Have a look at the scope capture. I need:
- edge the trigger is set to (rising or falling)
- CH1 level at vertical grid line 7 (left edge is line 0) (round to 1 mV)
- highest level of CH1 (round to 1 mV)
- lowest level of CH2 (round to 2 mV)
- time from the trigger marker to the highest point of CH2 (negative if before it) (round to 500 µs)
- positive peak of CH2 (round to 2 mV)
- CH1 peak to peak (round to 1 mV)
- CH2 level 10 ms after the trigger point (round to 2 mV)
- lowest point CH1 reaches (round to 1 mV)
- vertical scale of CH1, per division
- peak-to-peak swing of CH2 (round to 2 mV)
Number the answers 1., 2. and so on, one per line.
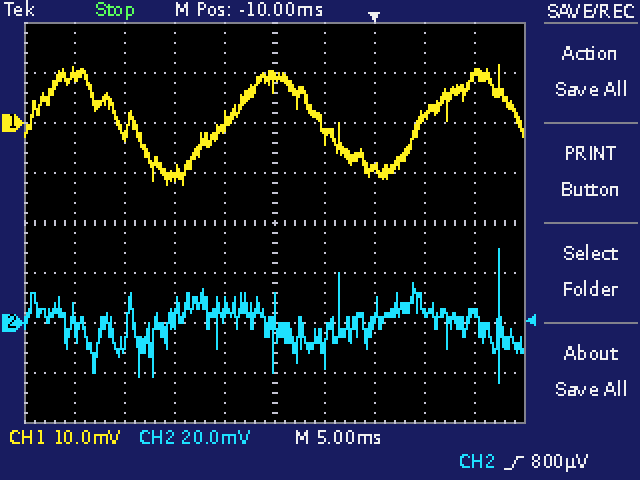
1. rising
2. -9 mV
3. 12 mV
4. -24 mV
5. +12.5 ms
6. 30 mV
7. 24 mV
8. 4 mV
9. -12 mV
10. 10 mV
11. 54 mV
